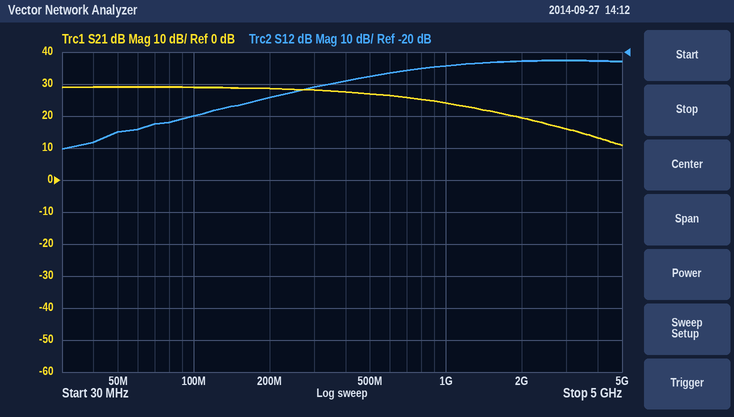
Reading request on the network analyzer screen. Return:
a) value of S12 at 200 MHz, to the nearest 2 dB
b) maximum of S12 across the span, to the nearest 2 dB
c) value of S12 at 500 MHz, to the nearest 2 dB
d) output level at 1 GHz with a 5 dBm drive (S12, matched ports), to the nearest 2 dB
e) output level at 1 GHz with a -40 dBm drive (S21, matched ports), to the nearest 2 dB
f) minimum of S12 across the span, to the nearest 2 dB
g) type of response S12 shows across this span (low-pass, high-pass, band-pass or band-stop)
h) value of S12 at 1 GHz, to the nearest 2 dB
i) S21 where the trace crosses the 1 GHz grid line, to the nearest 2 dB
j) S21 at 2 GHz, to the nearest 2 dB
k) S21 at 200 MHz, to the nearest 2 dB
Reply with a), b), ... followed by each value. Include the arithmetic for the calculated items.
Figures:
a) -34 dB
b) -22 dB
c) -28 dB
d) 5 dBm + (-24 dB) = -20 dBm
e) -40 dBm + (24 dB) = -16 dBm
f) -50 dB
g) high-pass
h) -24 dB
i) 24 dB
j) 20 dB
k) 28 dB
